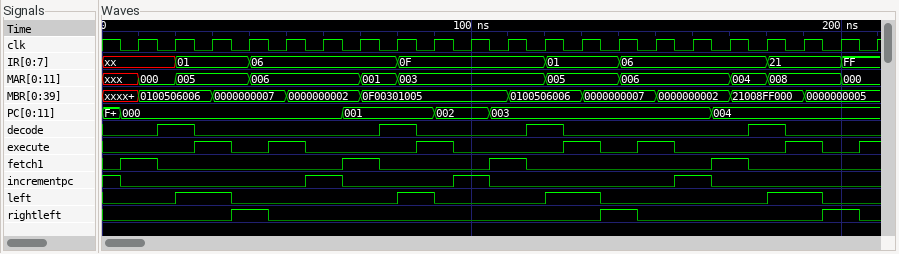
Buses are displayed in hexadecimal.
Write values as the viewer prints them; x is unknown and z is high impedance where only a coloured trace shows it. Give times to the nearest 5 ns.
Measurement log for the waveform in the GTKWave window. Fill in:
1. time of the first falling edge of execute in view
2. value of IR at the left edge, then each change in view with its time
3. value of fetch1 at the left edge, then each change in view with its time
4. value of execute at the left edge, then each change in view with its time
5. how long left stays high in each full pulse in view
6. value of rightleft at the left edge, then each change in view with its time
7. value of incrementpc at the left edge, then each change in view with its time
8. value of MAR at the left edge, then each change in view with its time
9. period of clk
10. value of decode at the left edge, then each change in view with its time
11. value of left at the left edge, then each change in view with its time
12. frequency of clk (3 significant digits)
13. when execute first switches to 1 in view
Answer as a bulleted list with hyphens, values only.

- 35 ns
- xx, 01 at 20 ns, 06 at 40 ns, 0F at 80 ns, 01 at 120 ns, 06 at 140 ns, 21 at 180 ns, FF at 200 ns
- 0, 1 at 5 ns, 0 at 15 ns, 1 at 65 ns, 0 at 75 ns, 1 at 105 ns, 0 at 115 ns, 1 at 165 ns, 0 at 175 ns
- 0, 1 at 25 ns, 0 at 35 ns, 1 at 45 ns, 0 at 55 ns, 1 at 85 ns, 0 at 95 ns, 1 at 125 ns, 0 at 135 ns, 1 at 145 ns, 0 at 155 ns, 1 at 185 ns, 0 at 195 ns, 1 at 205 ns
- 15 ns, 10 ns, 15 ns, 15 ns
- 0, 1 at 35 ns, 0 at 45 ns, 1 at 135 ns, 0 at 145 ns, 1 at 195 ns, 0 at 205 ns
- 1, 0 at 5 ns, 1 at 55 ns, 0 at 65 ns, 1 at 95 ns, 0 at 105 ns, 1 at 155 ns, 0 at 165 ns
- xxx, 000 at 10 ns, 005 at 20 ns, 006 at 40 ns, 001 at 70 ns, 003 at 80 ns, 005 at 120 ns, 006 at 140 ns, 004 at 170 ns, 008 at 180 ns, 000 at 200 ns
- 10 ns
- 0, 1 at 15 ns, 0 at 25 ns, 1 at 75 ns, 0 at 85 ns, 1 at 115 ns, 0 at 125 ns, 1 at 175 ns, 0 at 185 ns
- 0, 1 at 20 ns, 0 at 35 ns, 1 at 80 ns, 0 at 90 ns, 1 at 120 ns, 0 at 135 ns, 1 at 180 ns, 0 at 195 ns
- 100 MHz
- 25 ns
